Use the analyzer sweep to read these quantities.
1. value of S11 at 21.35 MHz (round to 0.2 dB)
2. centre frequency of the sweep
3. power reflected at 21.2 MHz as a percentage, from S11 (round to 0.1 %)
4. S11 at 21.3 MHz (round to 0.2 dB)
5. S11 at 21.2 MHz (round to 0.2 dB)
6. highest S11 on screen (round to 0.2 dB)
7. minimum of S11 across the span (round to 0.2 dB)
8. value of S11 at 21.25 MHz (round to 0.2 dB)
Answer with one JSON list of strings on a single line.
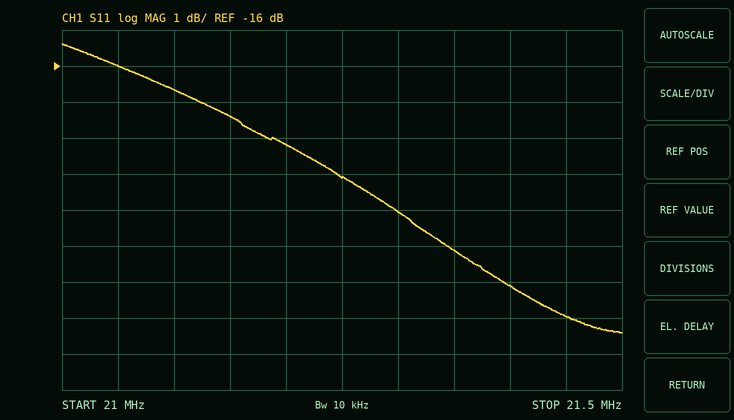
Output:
["-21.2 dB", "21.25 MHz", "1.5 %", "-20.0 dB", "-18.2 dB", "-15.4 dB", "-23.4 dB", "-19.0 dB"]
